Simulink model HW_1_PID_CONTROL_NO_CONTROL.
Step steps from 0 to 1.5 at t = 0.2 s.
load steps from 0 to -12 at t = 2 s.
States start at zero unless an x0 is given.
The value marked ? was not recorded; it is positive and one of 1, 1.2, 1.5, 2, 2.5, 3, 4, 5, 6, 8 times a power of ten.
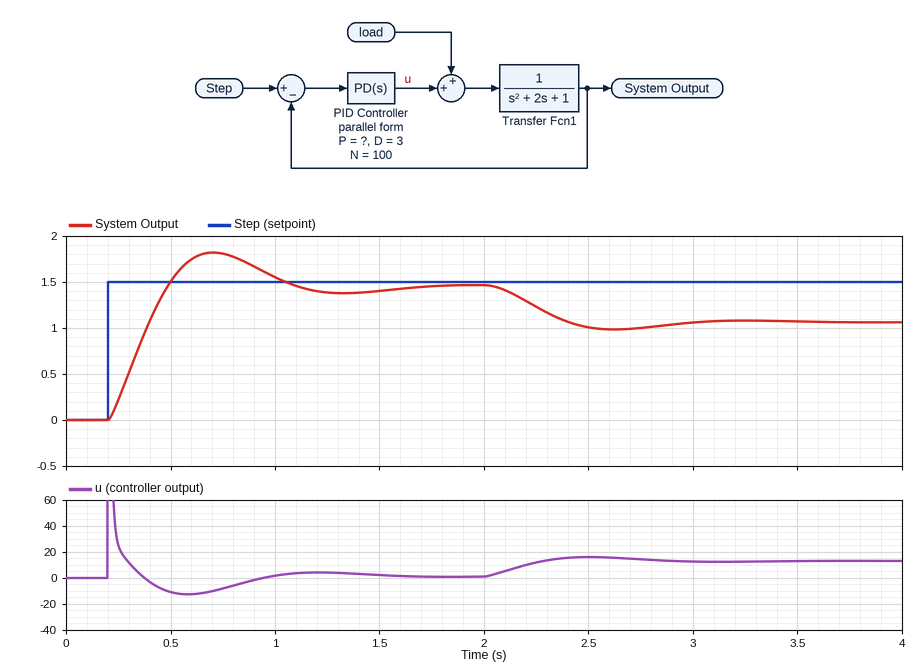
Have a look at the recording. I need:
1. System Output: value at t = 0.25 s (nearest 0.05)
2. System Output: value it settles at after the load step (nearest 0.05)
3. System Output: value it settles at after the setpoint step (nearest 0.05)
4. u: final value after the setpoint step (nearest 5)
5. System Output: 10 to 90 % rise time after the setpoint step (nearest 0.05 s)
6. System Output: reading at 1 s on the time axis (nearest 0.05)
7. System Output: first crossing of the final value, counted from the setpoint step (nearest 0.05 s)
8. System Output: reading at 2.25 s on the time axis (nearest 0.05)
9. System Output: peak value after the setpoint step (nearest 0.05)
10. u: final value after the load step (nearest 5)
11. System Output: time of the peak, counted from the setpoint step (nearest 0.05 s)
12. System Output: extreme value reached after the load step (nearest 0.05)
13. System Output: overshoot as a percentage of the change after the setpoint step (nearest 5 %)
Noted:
0.20
1.05
1.45
0
0.20 s
1.55
0.30 s
1.25
1.80
15
0.50 s
1.00
25 %
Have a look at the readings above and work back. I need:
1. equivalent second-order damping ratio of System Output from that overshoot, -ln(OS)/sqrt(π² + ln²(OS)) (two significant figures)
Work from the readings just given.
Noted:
0.40
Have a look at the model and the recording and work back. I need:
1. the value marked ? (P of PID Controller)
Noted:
30
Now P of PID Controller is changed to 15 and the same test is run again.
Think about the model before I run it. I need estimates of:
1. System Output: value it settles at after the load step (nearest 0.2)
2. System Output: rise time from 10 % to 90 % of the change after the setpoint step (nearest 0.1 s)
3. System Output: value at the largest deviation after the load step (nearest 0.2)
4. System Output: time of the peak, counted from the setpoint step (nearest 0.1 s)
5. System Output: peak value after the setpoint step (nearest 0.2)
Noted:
0.6
0.3 s
0.6
0.7 s
1.6
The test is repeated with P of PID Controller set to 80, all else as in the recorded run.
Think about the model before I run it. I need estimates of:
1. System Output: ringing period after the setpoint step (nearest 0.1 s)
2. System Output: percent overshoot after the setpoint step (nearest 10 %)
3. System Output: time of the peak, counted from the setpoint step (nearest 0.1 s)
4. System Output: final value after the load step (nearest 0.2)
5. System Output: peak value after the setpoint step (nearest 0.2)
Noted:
0.7 s
40 %
0.3 s
1.4
2.2
